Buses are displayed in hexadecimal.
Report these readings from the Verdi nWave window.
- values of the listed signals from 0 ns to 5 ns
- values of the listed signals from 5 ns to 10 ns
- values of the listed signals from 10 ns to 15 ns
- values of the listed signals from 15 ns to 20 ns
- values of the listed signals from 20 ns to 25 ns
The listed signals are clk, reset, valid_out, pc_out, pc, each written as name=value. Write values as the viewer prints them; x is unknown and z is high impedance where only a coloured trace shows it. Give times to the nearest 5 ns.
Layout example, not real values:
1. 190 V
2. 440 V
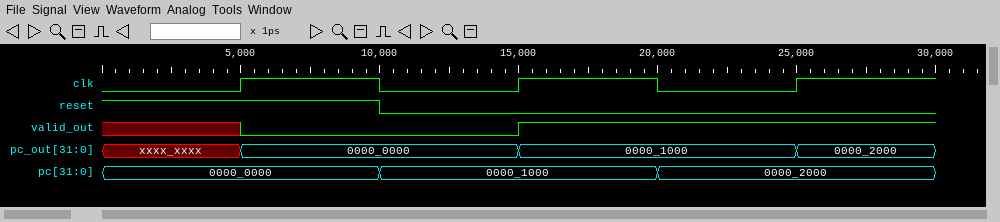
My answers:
1. clk=0, reset=1, valid_out=x, pc_out=xxxx_xxxx, pc=0000_0000
2. clk=1, reset=1, valid_out=0, pc_out=0000_0000, pc=0000_0000
3. clk=0, reset=0, valid_out=0, pc_out=0000_0000, pc=0000_1000
4. clk=1, reset=0, valid_out=1, pc_out=0000_1000, pc=0000_1000
5. clk=0, reset=0, valid_out=1, pc_out=0000_1000, pc=0000_2000
